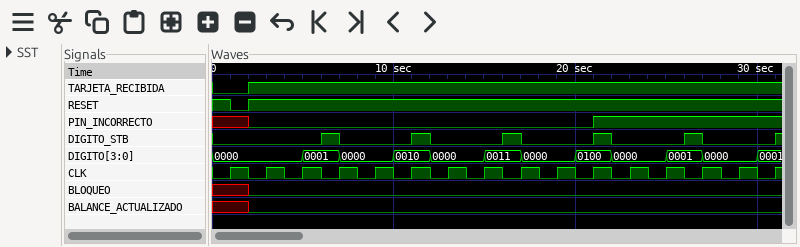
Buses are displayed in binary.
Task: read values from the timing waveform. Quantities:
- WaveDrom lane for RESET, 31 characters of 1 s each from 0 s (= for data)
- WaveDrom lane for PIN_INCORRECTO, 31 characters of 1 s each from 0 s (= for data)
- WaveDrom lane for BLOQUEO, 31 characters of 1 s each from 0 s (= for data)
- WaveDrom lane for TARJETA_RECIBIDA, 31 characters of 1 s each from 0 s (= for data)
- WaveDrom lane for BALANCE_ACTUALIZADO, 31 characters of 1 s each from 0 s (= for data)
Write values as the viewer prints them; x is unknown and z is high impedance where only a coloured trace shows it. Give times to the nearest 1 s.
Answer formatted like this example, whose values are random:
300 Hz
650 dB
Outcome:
{name: 'RESET', wave: '101............................'}
{name: 'PIN_INCORRECTO', wave: 'x.0..................1.........'}
{name: 'BLOQUEO', wave: 'x.0............................'}
{name: 'TARJETA_RECIBIDA', wave: '0.1............................'}
{name: 'BALANCE_ACTUALIZADO', wave: 'x.0............................'}
